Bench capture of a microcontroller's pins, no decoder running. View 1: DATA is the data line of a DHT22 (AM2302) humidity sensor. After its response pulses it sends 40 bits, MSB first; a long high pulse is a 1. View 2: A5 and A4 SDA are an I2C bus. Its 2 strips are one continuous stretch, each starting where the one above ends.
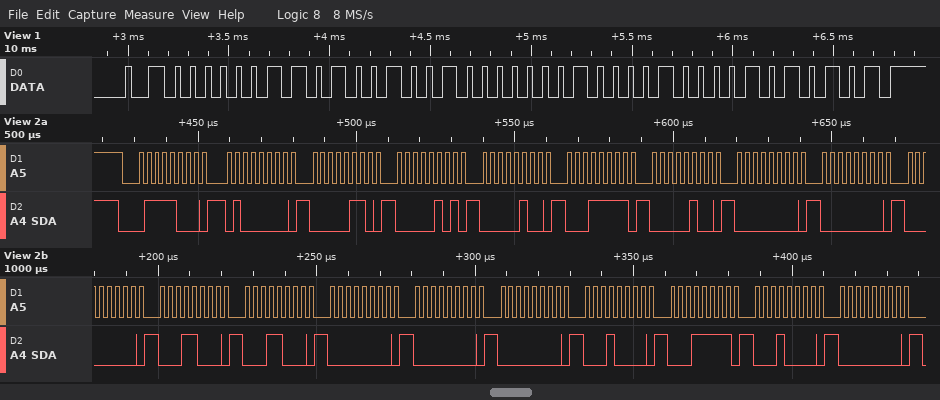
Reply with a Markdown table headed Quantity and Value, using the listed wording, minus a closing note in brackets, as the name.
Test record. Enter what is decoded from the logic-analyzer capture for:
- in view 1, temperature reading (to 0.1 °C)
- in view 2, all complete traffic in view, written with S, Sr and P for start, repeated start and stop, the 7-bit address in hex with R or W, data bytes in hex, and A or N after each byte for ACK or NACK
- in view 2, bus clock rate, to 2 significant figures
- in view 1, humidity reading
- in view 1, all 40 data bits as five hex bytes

| Quantity | Value |
|---|---|
| in view 1, temperature reading | 26.4 °C |
| in view 2, all complete traffic in view, written with S, Sr and P for start, repeated start and stop, the 7-bit address in hex with R or W, data bytes in hex, and A or N after each byte for ACK or NACK | S 3CW A 40 A 06 A 05 A 04 A 1F A 04 A 00 A 00 A 00 A 18 A 18 A 00 A 00 A 00 A 10 A 1F A 10 A 00 A |
| in view 2, bus clock rate, to 2 significant figures | 400 kHz |
| in view 1, humidity reading | 84.1 % |
| in view 1, all 40 data bits as five hex bytes | 03 49 01 08 55 |
